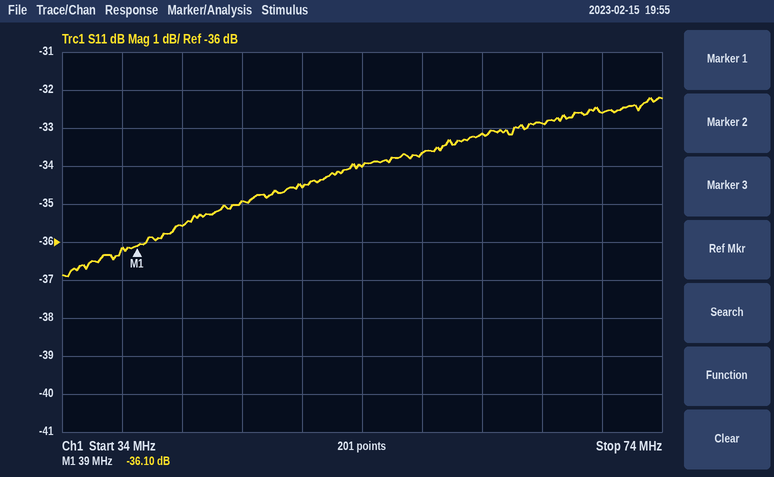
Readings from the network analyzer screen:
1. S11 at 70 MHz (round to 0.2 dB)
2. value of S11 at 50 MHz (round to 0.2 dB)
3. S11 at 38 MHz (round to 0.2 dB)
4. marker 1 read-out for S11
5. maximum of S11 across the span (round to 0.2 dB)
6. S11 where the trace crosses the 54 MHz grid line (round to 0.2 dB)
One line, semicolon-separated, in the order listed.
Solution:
-32.6 dB; -34.6 dB; -36.2 dB; -36.10 dB; -32.2 dB; -34.0 dB
